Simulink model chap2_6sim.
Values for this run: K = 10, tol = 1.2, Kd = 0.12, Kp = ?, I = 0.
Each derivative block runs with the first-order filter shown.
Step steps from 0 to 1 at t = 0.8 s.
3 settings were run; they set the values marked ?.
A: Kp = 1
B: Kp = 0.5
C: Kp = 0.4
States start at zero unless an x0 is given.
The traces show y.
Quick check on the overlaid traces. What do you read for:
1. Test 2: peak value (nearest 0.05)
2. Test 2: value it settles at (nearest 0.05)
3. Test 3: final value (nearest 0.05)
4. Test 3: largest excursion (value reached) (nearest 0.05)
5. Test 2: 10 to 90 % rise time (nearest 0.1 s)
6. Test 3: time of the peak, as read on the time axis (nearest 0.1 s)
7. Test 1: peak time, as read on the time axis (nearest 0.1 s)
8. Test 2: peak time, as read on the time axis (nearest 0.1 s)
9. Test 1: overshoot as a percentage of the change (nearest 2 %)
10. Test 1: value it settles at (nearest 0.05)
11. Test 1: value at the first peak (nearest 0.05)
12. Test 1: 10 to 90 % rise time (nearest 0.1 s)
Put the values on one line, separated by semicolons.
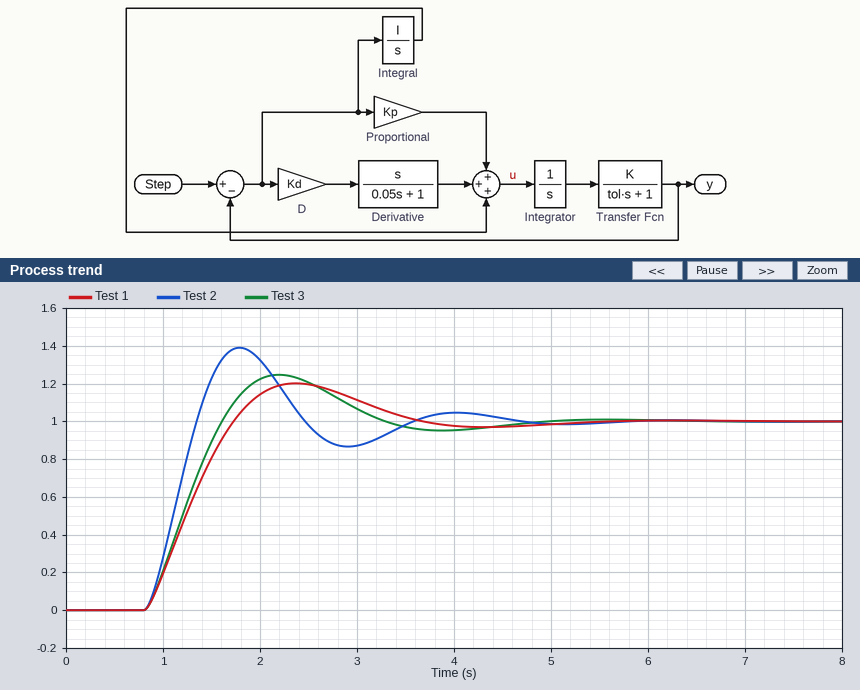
1.40; 1.00; 1.00; 1.25; 0.4 s; 2.2 s; 2.4 s; 1.8 s; 20 %; 1.00; 1.20; 0.7 s
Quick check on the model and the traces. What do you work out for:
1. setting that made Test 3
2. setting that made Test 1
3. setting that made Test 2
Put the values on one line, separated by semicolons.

B; C; A
